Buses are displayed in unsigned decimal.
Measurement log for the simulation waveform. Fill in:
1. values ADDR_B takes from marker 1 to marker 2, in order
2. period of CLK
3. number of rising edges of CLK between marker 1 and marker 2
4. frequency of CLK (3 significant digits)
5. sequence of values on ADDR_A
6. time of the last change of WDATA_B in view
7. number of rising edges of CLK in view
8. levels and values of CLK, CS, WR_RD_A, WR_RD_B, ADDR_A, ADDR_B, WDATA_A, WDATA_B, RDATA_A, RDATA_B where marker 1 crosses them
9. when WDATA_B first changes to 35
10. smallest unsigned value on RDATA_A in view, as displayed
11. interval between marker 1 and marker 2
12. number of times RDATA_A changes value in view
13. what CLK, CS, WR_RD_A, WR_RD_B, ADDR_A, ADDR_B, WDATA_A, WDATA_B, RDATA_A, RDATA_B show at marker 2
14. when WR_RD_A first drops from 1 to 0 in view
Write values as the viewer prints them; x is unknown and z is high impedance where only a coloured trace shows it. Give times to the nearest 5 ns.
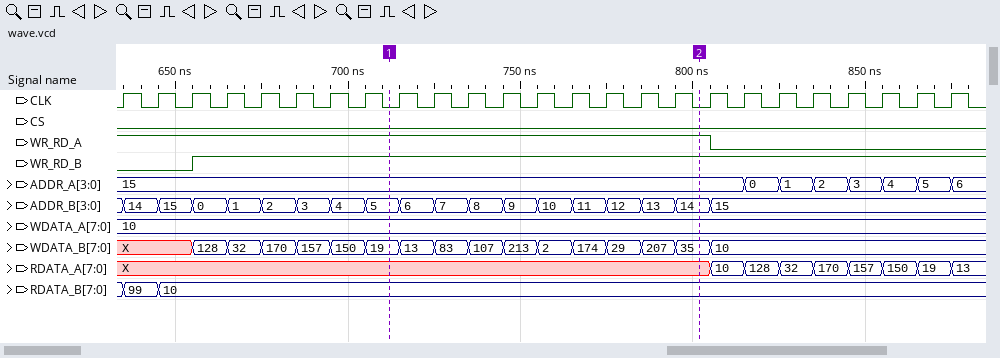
5, 6, 7, 8, 9, 10, 11, 12, 13, 14
10 ns
9
100 MHz
15, 0, 1, 2, 3, 4, 5, 6
805 ns
25
CLK=0, CS=0, WR_RD_A=1, WR_RD_B=1, ADDR_A=15, ADDR_B=5, WDATA_A=10, WDATA_B=19, RDATA_A=X, RDATA_B=10
795 ns
10
90 ns
8
CLK=0, CS=0, WR_RD_A=1, WR_RD_B=1, ADDR_A=15, ADDR_B=14, WDATA_A=10, WDATA_B=35, RDATA_A=X, RDATA_B=10
805 ns
